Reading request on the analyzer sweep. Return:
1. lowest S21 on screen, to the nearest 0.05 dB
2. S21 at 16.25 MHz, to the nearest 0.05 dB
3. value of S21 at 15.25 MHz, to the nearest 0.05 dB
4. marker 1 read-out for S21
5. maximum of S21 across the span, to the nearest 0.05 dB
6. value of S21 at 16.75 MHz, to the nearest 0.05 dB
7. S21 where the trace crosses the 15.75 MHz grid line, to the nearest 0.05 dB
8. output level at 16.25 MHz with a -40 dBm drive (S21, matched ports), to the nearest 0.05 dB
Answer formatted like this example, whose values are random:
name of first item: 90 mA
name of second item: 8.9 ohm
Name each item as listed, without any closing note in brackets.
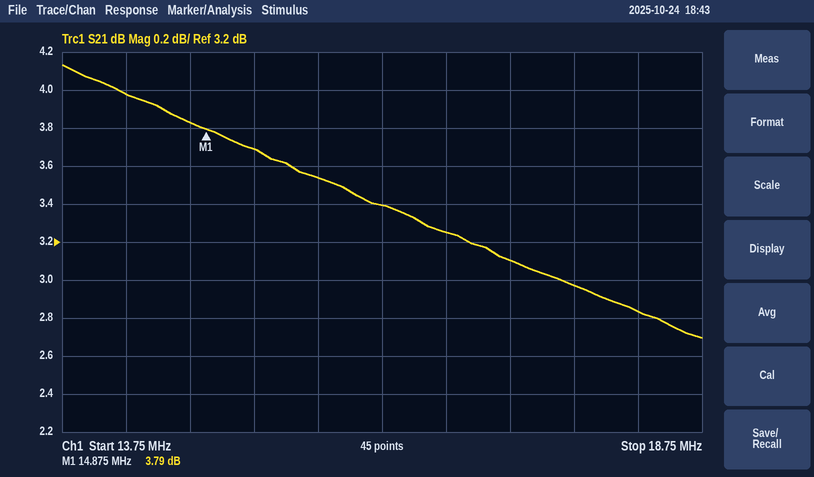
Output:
lowest S21 on screen, to the nearest 0.05 dB: 2.70 dB
S21 at 16.25 MHz, to the nearest 0.05 dB: 3.40 dB
value of S21 at 15.25 MHz, to the nearest 0.05 dB: 3.70 dB
marker 1 read-out for S21: 3.79 dB
maximum of S21 across the span, to the nearest 0.05 dB: 4.15 dB
value of S21 at 16.75 MHz, to the nearest 0.05 dB: 3.25 dB
S21 where the trace crosses the 15.75 MHz grid line, to the nearest 0.05 dB: 3.55 dB
output level at 16.25 MHz with a -40 dBm drive (S21, matched ports), to the nearest 0.05 dB: -36.60 dBm
